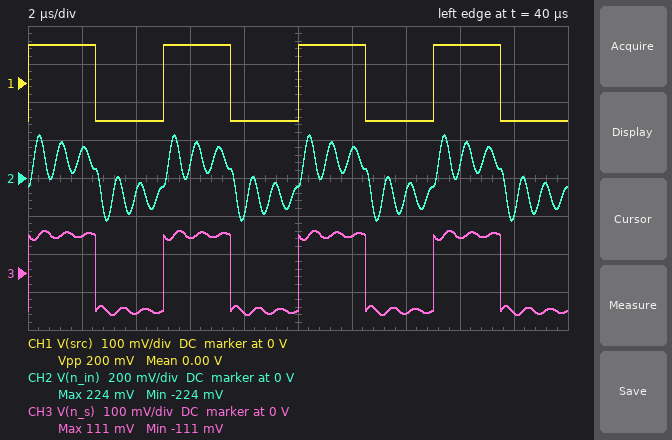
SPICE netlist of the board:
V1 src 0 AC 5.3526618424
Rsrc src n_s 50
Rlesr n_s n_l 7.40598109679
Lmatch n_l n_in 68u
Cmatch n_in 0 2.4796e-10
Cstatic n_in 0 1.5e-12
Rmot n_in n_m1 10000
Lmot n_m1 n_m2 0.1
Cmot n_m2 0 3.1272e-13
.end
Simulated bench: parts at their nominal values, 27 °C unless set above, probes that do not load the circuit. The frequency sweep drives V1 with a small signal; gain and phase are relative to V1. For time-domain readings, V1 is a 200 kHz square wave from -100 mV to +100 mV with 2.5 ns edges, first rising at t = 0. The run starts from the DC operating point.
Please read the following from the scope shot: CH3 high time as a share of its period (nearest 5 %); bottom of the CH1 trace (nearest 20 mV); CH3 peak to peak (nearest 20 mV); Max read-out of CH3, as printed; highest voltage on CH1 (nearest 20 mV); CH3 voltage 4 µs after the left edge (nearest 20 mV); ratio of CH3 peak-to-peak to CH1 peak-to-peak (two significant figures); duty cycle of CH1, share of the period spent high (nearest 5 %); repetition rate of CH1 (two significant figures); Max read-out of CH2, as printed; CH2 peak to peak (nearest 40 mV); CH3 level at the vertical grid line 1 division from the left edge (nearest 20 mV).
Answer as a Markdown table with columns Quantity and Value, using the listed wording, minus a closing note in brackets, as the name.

| Quantity | Value |
|---|---|
| CH3 high time as a share of its period | 50 % |
| bottom of the CH1 trace | -100 mV |
| CH3 peak to peak | 220 mV |
| Max read-out of CH3, as printed | 111 mV |
| highest voltage on CH1 | 100 mV |
| CH3 voltage 4 µs after the left edge | -100 mV |
| ratio of CH3 peak-to-peak to CH1 peak-to-peak | 1.1 |
| duty cycle of CH1, share of the period spent high | 50 % |
| repetition rate of CH1 | 200 kHz |
| Max read-out of CH2, as printed | 224 mV |
| CH2 peak to peak | 440 mV |
| CH3 level at the vertical grid line 1 division from the left edge | 100 mV |
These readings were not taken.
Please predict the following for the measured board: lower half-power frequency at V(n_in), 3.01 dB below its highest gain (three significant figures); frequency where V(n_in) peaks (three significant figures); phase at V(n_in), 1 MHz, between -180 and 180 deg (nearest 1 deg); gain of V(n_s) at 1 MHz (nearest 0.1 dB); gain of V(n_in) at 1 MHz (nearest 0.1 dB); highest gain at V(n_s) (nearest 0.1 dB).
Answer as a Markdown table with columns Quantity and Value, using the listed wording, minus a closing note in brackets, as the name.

| Quantity | Value |
|---|---|
| lower half-power frequency at V(n_in), 3.01 dB below its highest gain | 1.15 MHz |
| frequency where V(n_in) peaks | 1.22 MHz |
| phase at V(n_in), 1 MHz, between -180 and 180 deg | -15 deg |
| gain of V(n_s) at 1 MHz | -0.3 dB |
| gain of V(n_in) at 1 MHz | 9.2 dB |
| highest gain at V(n_s) | 0 dB |
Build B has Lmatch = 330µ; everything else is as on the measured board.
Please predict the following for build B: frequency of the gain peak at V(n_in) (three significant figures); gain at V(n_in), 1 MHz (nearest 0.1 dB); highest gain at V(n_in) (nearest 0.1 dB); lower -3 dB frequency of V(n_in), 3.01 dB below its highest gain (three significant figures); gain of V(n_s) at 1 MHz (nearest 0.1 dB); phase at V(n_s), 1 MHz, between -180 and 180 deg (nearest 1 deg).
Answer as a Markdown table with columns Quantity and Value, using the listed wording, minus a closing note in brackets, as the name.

| Quantity | Value |
|---|---|
| frequency of the gain peak at V(n_in) | 554 kHz |
| gain at V(n_in), 1 MHz | -7.0 dB |
| highest gain at V(n_in) | 26.0 dB |
| lower -3 dB frequency of V(n_in), 3.01 dB below its highest gain | 540 kHz |
| gain of V(n_s) at 1 MHz | 0 dB |
| phase at V(n_s), 1 MHz, between -180 and 180 deg | 2 deg |
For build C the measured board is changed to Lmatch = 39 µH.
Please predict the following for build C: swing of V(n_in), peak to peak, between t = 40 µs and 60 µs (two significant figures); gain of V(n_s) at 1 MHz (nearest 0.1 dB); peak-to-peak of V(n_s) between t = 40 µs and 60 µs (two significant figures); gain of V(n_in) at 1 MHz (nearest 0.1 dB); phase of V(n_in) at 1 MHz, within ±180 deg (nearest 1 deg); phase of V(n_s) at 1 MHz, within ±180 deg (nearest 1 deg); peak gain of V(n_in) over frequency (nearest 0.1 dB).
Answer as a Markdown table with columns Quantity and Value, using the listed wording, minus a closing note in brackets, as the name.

| Quantity | Value |
|---|---|
| swing of V(n_in), peak to peak, between t = 40 µs and 60 µs | 470 mV |
| gain of V(n_s) at 1 MHz | -0.1 dB |
| peak-to-peak of V(n_s) between t = 40 µs and 60 µs | 230 mV |
| gain of V(n_in) at 1 MHz | 4.1 dB |
| phase of V(n_in) at 1 MHz, within ±180 deg | -8 deg |
| phase of V(n_s) at 1 MHz, within ±180 deg | -7 deg |
| peak gain of V(n_in) over frequency | 16.8 dB |
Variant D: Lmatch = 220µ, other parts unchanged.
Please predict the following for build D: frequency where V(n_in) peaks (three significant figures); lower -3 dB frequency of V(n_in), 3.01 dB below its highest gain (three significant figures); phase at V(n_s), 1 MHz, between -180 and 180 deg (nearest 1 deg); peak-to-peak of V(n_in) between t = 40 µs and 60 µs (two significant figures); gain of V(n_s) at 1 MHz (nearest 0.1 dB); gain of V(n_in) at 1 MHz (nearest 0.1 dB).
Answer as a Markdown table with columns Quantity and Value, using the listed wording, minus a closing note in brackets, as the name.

| Quantity | Value |
|---|---|
| frequency where V(n_in) peaks | 678 kHz |
| lower -3 dB frequency of V(n_in), 3.01 dB below its highest gain | 657 kHz |
| phase at V(n_s), 1 MHz, between -180 and 180 deg | 4 deg |
| peak-to-peak of V(n_in) between t = 40 µs and 60 µs | 570 mV |
| gain of V(n_s) at 1 MHz | 0 dB |
| gain of V(n_in) at 1 MHz | -1.3 dB |
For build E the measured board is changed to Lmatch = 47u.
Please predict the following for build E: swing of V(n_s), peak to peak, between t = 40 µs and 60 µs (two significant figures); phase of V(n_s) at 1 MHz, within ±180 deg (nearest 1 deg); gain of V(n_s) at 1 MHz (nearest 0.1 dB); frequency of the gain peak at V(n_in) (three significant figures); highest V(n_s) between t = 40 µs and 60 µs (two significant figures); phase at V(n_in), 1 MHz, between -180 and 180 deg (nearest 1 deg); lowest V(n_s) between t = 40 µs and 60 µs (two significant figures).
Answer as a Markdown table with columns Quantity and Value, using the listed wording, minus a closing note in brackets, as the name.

| Quantity | Value |
|---|---|
| swing of V(n_s), peak to peak, between t = 40 µs and 60 µs | 240 mV |
| phase of V(n_s) at 1 MHz, within ±180 deg | -8 deg |
| gain of V(n_s) at 1 MHz | -0.1 dB |
| frequency of the gain peak at V(n_in) | 1.46 MHz |
| highest V(n_s) between t = 40 µs and 60 µs | 120 mV |
| phase at V(n_in), 1 MHz, between -180 and 180 deg | -9 deg |
| lowest V(n_s) between t = 40 µs and 60 µs | -120 mV |
